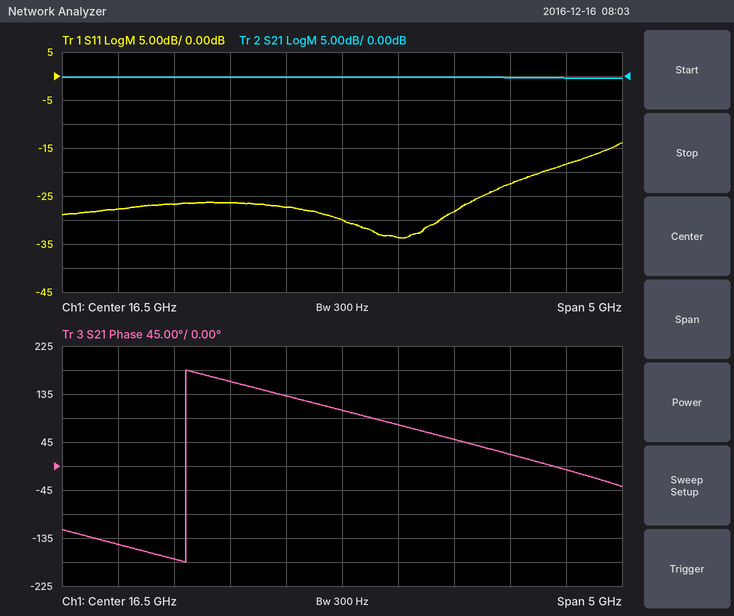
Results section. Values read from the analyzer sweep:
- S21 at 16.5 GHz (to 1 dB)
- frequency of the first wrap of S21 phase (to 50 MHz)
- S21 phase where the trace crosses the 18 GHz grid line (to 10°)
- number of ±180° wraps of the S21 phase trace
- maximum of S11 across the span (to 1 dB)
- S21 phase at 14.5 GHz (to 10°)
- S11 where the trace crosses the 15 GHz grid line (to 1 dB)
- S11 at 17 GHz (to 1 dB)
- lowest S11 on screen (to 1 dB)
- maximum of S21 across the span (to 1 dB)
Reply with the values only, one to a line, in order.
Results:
0 dB
15.10 GHz
20°
1
-14 dB
-150°
-27 dB
-34 dB
-34 dB
0 dB
